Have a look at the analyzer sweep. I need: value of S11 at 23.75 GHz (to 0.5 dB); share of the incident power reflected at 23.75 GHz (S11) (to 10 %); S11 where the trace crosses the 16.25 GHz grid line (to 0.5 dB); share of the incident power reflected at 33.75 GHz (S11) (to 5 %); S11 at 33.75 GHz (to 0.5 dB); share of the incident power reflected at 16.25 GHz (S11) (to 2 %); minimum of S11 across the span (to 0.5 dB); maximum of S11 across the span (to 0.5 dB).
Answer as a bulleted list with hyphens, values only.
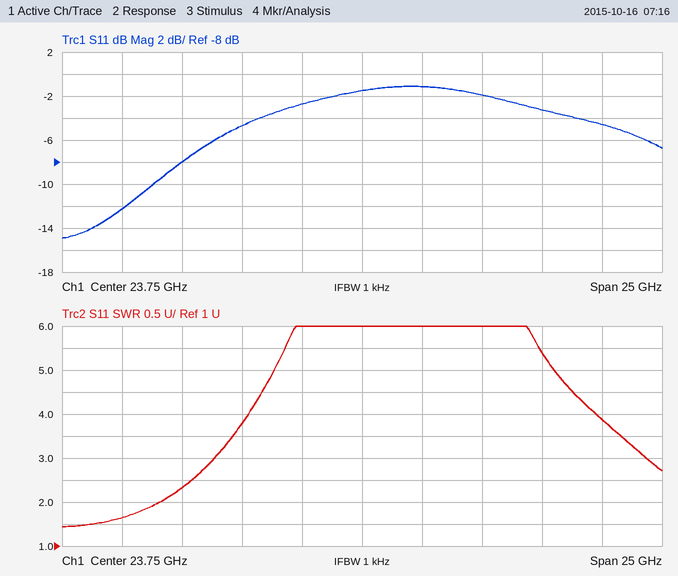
- -1.5 dB
- 70 %
- -8.0 dB
- 35 %
- -4.5 dB
- 16 %
- -15.0 dB
- -1.0 dB
